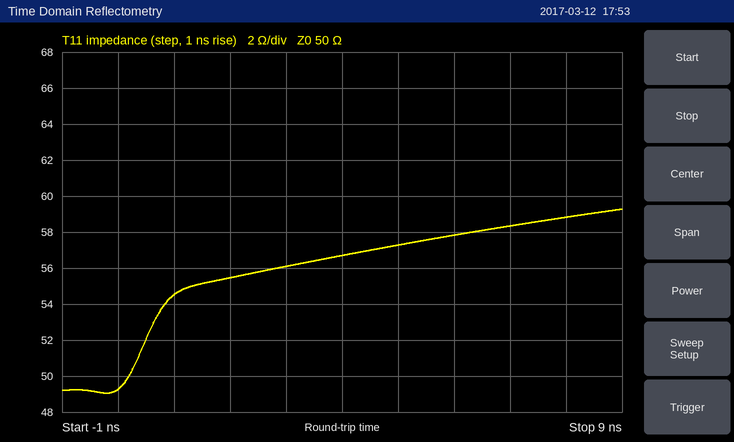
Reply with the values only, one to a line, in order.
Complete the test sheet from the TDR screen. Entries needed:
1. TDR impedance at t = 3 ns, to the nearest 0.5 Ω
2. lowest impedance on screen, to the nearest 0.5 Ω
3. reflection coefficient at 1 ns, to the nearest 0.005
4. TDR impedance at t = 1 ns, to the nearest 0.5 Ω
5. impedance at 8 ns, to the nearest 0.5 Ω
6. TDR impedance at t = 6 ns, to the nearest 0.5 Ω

56.0 Ω
49.0 Ω
+0.045
54.5 Ω
59.0 Ω
58.0 Ω
